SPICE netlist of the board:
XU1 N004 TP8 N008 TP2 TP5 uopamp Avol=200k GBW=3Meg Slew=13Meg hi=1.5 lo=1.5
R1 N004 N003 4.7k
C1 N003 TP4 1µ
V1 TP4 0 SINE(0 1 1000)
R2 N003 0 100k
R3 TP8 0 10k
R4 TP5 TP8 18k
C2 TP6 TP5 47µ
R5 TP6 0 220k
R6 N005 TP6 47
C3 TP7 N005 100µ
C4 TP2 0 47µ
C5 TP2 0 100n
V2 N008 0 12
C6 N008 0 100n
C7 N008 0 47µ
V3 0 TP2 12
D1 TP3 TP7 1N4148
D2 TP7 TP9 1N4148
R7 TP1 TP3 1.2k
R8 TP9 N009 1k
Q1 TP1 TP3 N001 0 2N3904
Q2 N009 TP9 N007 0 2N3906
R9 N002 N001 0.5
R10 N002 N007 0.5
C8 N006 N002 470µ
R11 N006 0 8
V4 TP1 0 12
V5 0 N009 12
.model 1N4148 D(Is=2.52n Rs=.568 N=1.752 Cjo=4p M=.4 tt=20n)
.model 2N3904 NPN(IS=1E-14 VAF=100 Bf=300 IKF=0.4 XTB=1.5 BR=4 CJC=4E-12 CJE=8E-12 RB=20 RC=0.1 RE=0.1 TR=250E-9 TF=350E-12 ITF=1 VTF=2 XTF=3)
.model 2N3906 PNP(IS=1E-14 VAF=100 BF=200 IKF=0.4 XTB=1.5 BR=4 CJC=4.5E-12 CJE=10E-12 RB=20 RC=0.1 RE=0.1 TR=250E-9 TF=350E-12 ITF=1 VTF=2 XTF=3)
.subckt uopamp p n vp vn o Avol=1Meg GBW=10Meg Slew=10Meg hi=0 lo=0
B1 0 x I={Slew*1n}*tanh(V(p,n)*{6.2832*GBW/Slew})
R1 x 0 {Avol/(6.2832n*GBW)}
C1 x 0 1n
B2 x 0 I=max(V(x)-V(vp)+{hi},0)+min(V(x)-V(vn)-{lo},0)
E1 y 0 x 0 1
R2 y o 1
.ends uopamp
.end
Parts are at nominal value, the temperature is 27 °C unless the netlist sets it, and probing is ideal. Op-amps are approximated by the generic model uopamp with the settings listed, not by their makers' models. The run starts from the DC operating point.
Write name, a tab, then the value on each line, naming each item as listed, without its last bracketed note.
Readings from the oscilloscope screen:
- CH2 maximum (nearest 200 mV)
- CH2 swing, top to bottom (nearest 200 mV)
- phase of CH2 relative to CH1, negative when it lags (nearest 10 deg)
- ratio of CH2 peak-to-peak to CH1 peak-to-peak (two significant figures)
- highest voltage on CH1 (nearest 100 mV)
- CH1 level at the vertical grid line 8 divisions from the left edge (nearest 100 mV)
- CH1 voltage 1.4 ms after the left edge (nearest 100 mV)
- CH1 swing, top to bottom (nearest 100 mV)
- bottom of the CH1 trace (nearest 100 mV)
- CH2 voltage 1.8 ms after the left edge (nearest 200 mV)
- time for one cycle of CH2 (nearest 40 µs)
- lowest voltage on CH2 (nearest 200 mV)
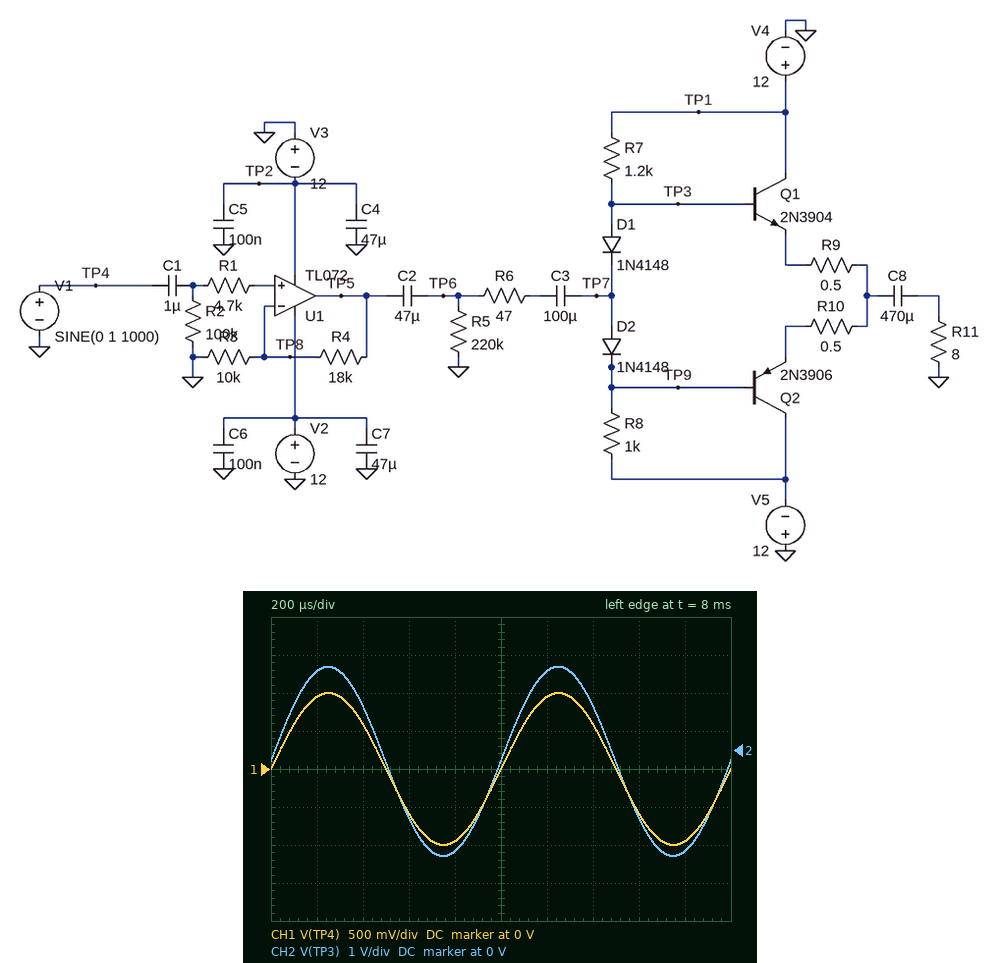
CH2 maximum	2.2 V
CH2 swing, top to bottom	5.0 V
phase of CH2 relative to CH1, negative when it lags	0 deg
ratio of CH2 peak-to-peak to CH1 peak-to-peak	2.5
highest voltage on CH1	1.0 V
CH1 level at the vertical grid line 8 divisions from the left edge	-600 mV
CH1 voltage 1.4 ms after the left edge	600 mV
CH1 swing, top to bottom	2.0 V
bottom of the CH1 trace	-1.0 V
CH2 voltage 1.8 ms after the left edge	-2.6 V
time for one cycle of CH2	1.00 ms
lowest voltage on CH2	-2.8 V
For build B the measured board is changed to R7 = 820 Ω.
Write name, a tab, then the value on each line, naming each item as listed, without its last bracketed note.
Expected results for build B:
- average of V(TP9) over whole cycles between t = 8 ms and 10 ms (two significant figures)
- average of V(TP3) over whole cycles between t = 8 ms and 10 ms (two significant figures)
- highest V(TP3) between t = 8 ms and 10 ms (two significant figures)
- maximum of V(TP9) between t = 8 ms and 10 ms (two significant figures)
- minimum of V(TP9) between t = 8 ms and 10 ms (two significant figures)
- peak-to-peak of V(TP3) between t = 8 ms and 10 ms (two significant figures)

average of V(TP9) over whole cycles between t = 8 ms and 10 ms	440 mV
average of V(TP3) over whole cycles between t = 8 ms and 10 ms	1.8 V
highest V(TP3) between t = 8 ms and 10 ms	4.3 V
maximum of V(TP9) between t = 8 ms and 10 ms	2.9 V
minimum of V(TP9) between t = 8 ms and 10 ms	-2.0 V
peak-to-peak of V(TP3) between t = 8 ms and 10 ms	4.9 V
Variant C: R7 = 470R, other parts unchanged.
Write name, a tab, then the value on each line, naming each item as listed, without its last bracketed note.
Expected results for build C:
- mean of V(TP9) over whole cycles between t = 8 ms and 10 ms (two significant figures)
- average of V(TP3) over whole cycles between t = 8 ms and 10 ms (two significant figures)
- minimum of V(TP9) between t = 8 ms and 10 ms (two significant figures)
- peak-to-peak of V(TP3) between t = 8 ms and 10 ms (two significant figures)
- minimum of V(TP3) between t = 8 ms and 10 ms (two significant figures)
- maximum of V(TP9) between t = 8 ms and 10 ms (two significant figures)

mean of V(TP9) over whole cycles between t = 8 ms and 10 ms	3.4 V
average of V(TP3) over whole cycles between t = 8 ms and 10 ms	4.8 V
minimum of V(TP9) between t = 8 ms and 10 ms	1.0 V
peak-to-peak of V(TP3) between t = 8 ms and 10 ms	4.7 V
minimum of V(TP3) between t = 8 ms and 10 ms	2.4 V
maximum of V(TP9) between t = 8 ms and 10 ms	5.7 V
